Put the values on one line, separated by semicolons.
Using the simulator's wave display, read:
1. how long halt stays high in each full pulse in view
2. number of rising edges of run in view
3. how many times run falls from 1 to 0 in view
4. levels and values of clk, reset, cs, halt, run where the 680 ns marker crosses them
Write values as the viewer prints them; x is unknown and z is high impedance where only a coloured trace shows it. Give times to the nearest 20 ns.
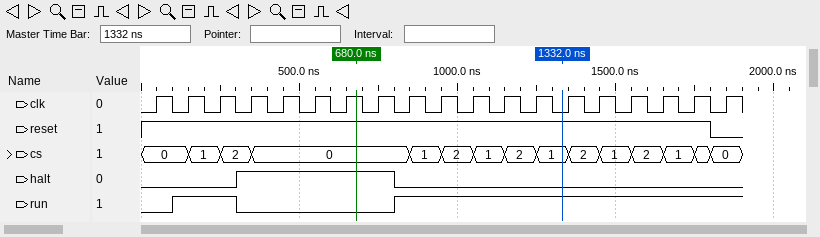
500 ns; 2; 1; clk=1, reset=1, cs=0, halt=1, run=0
